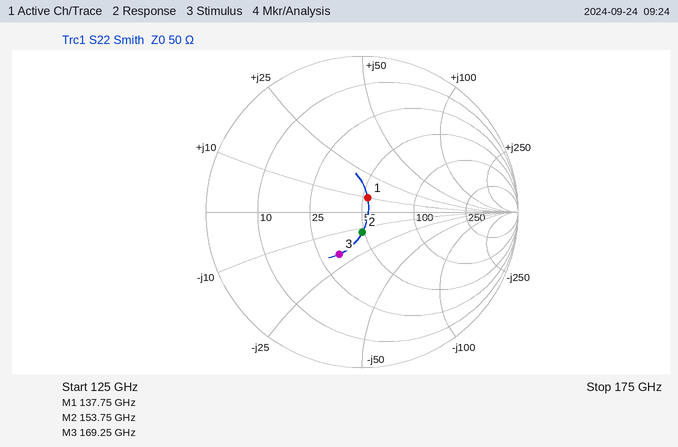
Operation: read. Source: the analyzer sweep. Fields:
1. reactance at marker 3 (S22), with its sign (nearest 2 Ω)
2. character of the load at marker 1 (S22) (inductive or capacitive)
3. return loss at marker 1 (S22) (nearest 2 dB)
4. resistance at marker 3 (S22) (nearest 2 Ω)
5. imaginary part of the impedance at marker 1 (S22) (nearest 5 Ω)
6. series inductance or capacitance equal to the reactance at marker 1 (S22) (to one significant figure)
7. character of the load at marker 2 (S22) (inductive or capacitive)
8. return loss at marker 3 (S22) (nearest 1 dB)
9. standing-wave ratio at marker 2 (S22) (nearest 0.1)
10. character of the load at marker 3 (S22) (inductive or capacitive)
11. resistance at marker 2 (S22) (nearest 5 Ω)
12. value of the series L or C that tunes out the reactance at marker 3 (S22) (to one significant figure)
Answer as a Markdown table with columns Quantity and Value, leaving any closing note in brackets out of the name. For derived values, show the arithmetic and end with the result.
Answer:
| Quantity | Value |
|---|---|
| reactance at marker 3 (S22), with its sign | -20 Ω |
| character of the load at marker 1 (S22) | inductive |
| return loss at marker 1 (S22) | 20 dB |
| resistance at marker 3 (S22) | 32 Ω |
| imaginary part of the impedance at marker 1 (S22) | +10 Ω |
| series inductance or capacitance equal to the reactance at marker 1 (S22) | L = 10 Ω/(2π × 137.75 GHz) ≈ 11.6 pH, so 10 pH to one significant figure |
| character of the load at marker 2 (S22) | capacitive |
| return loss at marker 3 (S22) | 10 dB |
| standing-wave ratio at marker 2 (S22) | 1.3 |
| character of the load at marker 3 (S22) | capacitive |
| resistance at marker 2 (S22) | 50 Ω |
| value of the series L or C that tunes out the reactance at marker 3 (S22) | L = 20 Ω/(2π × 169.25 GHz) ≈ 18.8 pH, so 20 pH to one significant figure |
